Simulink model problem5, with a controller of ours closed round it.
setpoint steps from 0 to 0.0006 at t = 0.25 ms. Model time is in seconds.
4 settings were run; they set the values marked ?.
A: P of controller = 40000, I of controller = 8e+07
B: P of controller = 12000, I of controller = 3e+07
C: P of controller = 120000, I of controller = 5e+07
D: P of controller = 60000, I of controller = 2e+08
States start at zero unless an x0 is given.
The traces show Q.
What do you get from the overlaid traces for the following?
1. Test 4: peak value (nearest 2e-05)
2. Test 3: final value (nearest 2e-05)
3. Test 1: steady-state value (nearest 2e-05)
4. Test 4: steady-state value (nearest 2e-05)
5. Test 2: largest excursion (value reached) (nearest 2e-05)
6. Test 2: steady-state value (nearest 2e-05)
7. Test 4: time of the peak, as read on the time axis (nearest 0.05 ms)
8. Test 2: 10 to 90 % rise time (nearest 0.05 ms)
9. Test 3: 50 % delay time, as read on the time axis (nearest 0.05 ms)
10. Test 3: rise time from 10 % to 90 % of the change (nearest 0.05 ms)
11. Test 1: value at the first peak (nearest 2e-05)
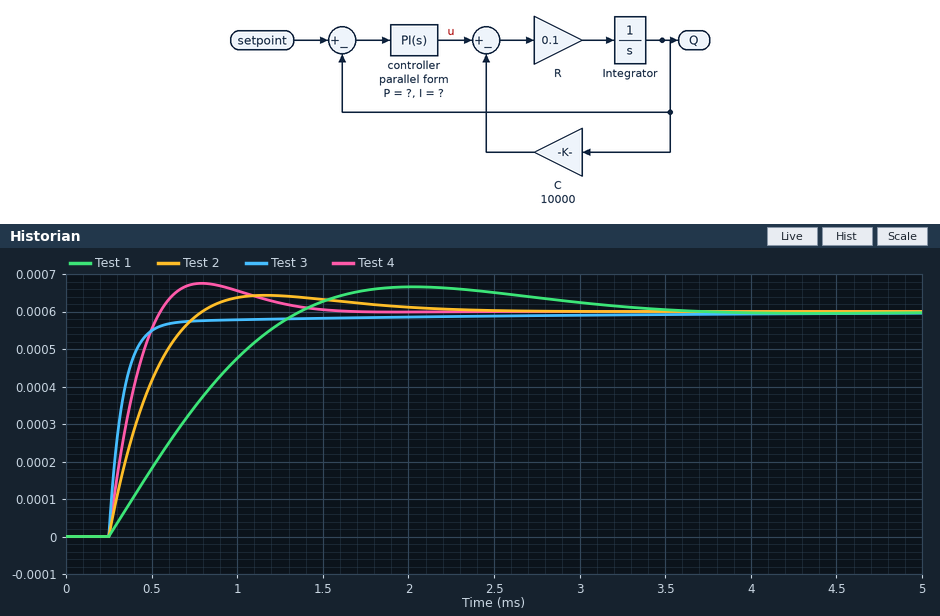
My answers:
0.00068
0.00060
0.00060
0.00060
0.00064
0.00060
0.80 ms
0.40 ms
0.30 ms
0.20 ms
0.00066
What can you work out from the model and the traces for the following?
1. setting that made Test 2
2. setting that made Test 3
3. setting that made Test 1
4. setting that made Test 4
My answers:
A
C
B
D
